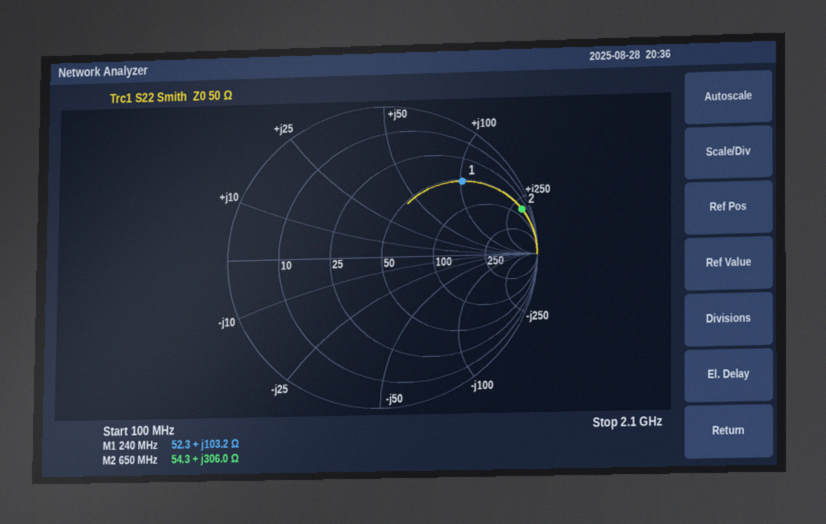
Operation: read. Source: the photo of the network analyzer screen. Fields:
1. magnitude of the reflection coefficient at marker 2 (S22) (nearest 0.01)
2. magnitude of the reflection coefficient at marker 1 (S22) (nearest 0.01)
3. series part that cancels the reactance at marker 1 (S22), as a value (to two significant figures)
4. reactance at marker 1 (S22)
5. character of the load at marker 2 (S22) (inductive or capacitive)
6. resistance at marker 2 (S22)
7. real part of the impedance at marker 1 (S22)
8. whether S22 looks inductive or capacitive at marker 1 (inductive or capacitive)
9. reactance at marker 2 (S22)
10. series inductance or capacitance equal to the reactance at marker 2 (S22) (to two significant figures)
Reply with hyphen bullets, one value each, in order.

- 0.95
- 0.71
- 6.4 pF
- +103.2 Ω
- inductive
- 54.3 Ω
- 52.3 Ω
- inductive
- +306.0 Ω
- 75 nH
